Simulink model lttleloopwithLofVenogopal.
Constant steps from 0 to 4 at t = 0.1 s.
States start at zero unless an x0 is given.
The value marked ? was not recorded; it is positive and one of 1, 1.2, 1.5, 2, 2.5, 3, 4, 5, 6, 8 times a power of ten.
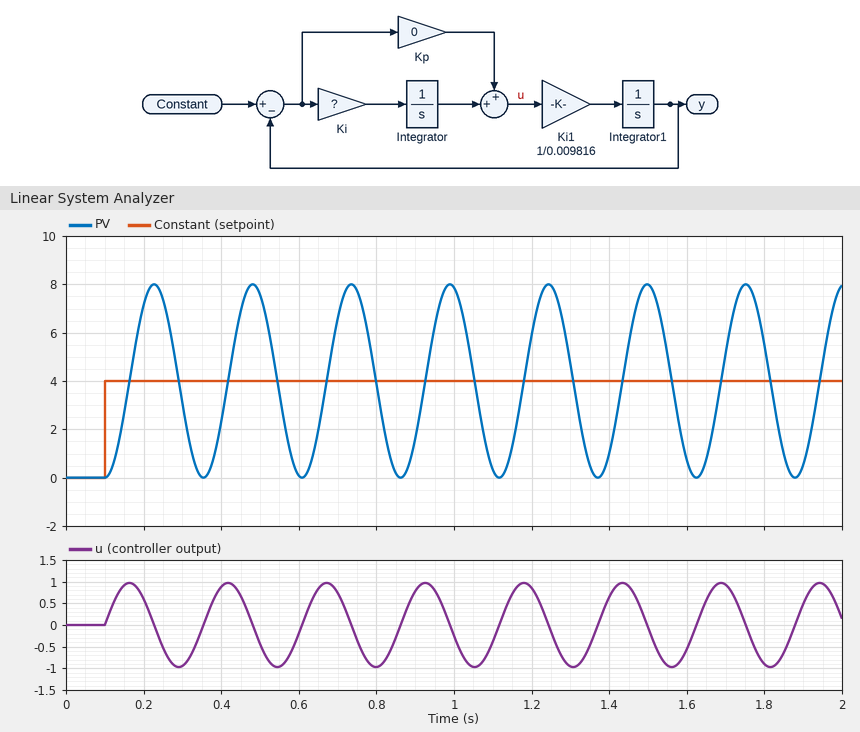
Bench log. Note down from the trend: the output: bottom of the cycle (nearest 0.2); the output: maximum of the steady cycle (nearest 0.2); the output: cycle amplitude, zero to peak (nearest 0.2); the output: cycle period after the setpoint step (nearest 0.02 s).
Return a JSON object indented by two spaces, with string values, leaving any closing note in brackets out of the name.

{
  "the output: bottom of the cycle": "0.0",
  "the output: maximum of the steady cycle": "8.0",
  "the output: cycle amplitude, zero to peak": "4.0",
  "the output: cycle period after the setpoint step": "0.26 s"
}
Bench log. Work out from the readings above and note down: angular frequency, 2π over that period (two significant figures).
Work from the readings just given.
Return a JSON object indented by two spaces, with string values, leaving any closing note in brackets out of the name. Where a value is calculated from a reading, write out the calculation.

{
  "angular frequency, 2π over that period": "2π / 0.26 = 24 rad/s"
}
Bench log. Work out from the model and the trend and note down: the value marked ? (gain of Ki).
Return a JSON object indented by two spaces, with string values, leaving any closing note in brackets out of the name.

{
  "the value marked ?": "6"
}
